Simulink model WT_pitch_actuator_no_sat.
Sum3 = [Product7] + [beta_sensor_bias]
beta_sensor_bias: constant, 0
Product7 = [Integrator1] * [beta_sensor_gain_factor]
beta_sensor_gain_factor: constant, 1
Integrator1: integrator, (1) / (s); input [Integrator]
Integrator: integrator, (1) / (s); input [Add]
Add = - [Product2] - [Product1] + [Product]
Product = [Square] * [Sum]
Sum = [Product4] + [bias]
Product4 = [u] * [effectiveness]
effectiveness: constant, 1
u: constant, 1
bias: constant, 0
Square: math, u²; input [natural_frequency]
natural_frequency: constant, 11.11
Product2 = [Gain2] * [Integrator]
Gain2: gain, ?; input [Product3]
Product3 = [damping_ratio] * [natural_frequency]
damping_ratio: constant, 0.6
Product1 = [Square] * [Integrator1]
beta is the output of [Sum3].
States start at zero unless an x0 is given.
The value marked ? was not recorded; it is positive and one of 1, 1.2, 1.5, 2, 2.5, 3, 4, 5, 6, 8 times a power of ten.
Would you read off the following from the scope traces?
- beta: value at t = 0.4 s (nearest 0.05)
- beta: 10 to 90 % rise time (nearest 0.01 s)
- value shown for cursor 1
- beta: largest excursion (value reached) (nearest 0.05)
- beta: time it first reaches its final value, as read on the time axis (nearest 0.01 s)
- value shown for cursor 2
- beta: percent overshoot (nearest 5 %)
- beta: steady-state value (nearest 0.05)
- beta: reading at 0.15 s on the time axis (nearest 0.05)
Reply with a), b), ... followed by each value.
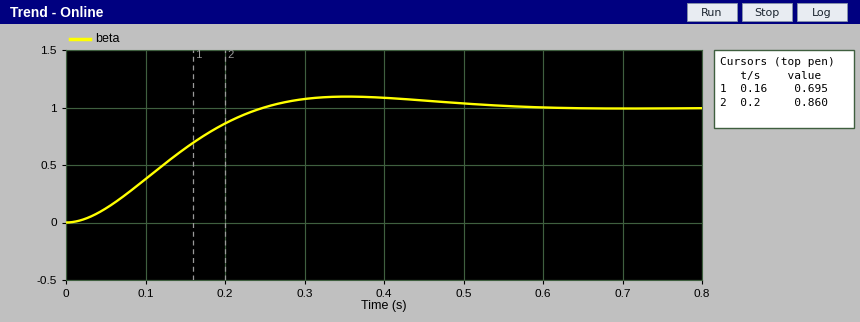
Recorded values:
a) 1.10
b) 0.17 s
c) 0.695
d) 1.10
e) 0.25 s
f) 0.860
g) 10 %
h) 1.00
i) 0.65
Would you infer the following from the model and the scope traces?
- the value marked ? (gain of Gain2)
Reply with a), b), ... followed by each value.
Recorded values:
a) 2
